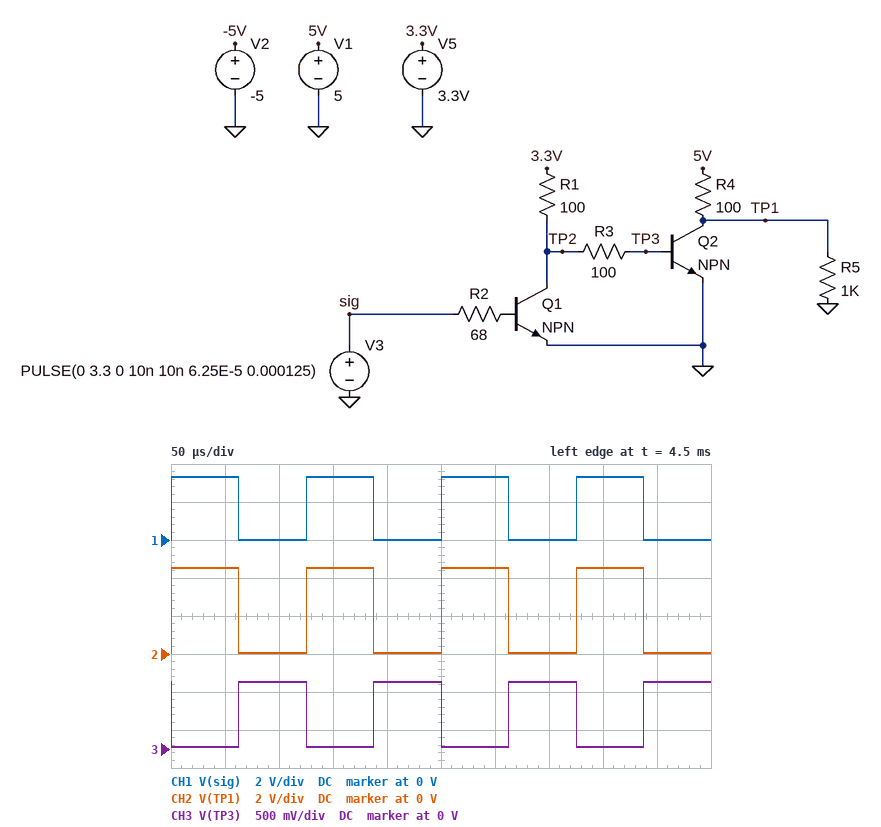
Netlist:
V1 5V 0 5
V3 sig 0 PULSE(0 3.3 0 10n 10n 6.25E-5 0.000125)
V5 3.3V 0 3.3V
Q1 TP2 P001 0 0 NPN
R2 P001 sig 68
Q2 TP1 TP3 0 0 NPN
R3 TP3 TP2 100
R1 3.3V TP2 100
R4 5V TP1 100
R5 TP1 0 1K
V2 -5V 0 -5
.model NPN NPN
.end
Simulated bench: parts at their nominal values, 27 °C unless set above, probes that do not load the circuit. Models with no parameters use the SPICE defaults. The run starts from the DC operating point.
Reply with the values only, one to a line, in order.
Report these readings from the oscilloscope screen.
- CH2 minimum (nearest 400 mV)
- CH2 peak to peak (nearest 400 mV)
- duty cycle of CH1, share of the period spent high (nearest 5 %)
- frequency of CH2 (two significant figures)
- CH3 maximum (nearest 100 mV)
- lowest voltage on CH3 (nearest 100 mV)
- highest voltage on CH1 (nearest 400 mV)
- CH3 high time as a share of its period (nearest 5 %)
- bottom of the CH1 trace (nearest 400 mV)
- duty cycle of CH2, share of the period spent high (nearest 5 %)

0 V
4.4 V
50 %
8.0 kHz
900 mV
0 V
3.2 V
50 %
0 V
50 %
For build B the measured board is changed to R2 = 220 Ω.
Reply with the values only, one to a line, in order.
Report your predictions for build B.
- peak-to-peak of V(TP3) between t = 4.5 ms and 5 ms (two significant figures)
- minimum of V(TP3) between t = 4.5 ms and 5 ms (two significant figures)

840 mV
42 mV
